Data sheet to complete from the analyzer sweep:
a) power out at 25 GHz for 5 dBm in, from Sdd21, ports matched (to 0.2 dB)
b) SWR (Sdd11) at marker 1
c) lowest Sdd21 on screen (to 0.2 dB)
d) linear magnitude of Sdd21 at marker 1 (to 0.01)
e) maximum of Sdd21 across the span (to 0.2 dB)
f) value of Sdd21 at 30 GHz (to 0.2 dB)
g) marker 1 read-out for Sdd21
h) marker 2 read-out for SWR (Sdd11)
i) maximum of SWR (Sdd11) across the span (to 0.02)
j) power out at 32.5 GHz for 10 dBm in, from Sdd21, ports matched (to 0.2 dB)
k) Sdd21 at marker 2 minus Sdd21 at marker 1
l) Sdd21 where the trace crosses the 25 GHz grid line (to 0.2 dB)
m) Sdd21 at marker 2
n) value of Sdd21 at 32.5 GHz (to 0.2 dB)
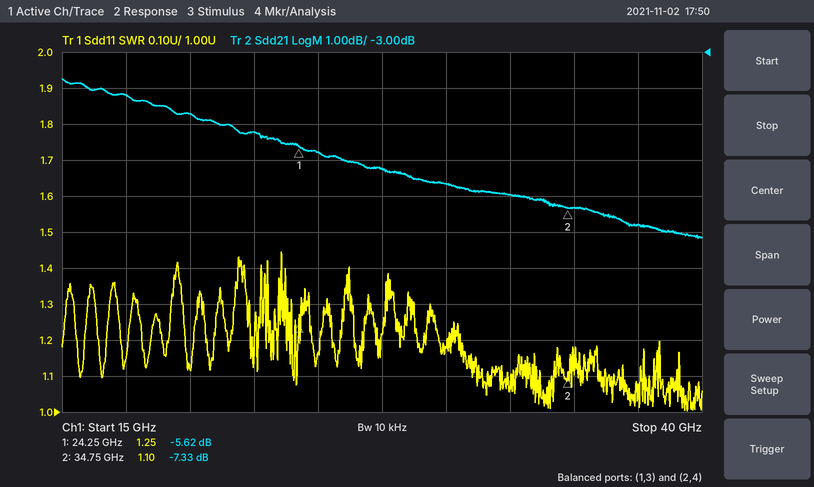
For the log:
-0.8 dBm
1.25
-8.2 dB
0.52
-3.8 dB
-6.6 dB
-5.62 dB
1.10
1.44
3.0 dBm
-1.71 dB
-5.8 dB
-7.33 dB
-7.0 dB
